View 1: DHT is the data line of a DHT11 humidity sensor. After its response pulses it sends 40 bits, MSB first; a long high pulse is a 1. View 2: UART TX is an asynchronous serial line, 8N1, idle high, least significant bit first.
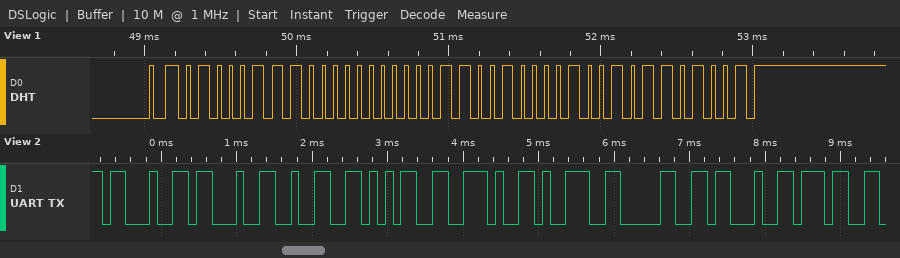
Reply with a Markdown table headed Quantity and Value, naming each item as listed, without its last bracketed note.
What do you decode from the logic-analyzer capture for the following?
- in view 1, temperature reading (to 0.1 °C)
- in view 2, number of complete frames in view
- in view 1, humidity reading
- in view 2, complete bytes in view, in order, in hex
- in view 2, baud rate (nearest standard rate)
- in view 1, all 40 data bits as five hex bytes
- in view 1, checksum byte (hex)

| Quantity | Value |
|---|---|
| in view 1, temperature reading | 25.9 °C |
| in view 2, number of complete frames in view | 9 |
| in view 1, humidity reading | 71 % |
| in view 2, complete bytes in view, in order, in hex | 23 23 32 35 2E 39 30 23 37 |
| in view 2, baud rate | 9600 baud |
| in view 1, all 40 data bits as five hex bytes | 47 00 19 09 69 |
| in view 1, checksum byte | 0x69 |
